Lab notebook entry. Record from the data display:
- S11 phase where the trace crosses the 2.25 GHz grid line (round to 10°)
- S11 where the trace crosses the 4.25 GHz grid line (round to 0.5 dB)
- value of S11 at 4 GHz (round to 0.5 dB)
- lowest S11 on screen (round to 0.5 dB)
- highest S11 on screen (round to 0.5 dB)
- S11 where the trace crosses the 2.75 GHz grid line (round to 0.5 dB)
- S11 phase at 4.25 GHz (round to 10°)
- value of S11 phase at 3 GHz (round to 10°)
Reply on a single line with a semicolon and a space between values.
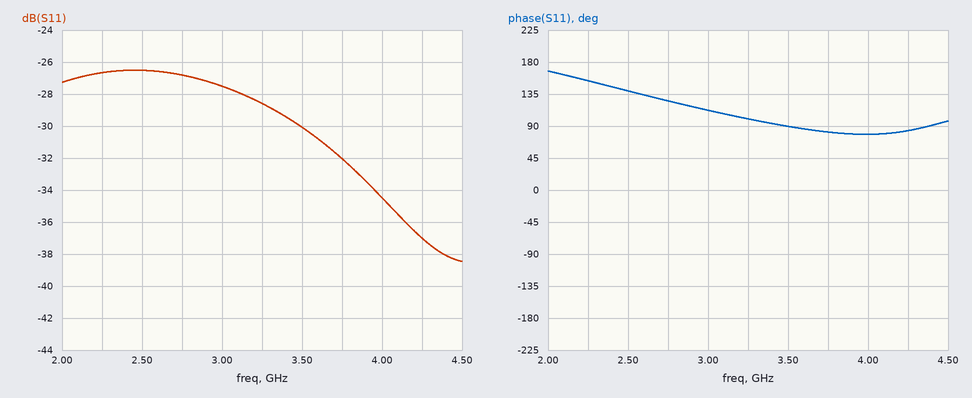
150°; -37.0 dB; -34.5 dB; -38.5 dB; -26.5 dB; -27.0 dB; 80°; 110°
